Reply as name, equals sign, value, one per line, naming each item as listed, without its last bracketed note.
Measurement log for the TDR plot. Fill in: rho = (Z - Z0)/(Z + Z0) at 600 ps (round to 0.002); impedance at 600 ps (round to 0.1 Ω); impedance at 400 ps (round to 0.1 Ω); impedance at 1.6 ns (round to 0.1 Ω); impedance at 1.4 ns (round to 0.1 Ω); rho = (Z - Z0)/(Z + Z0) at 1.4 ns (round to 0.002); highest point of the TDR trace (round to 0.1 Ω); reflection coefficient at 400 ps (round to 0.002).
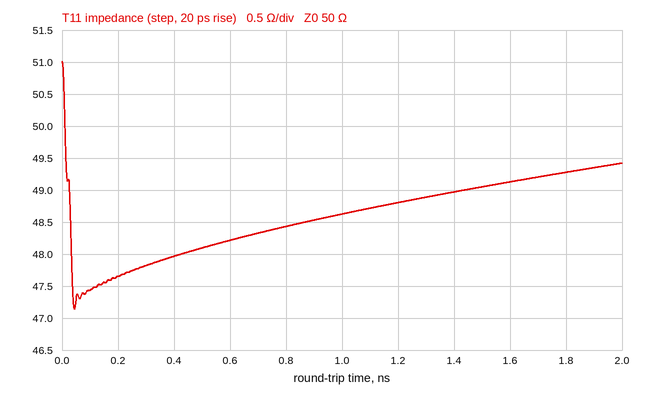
rho = (Z - Z0)/(Z + Z0) at 600 ps = -0.018
impedance at 600 ps = 48.2 Ω
impedance at 400 ps = 48.0 Ω
impedance at 1.6 ns = 49.1 Ω
impedance at 1.4 ns = 49.0 Ω
rho = (Z - Z0)/(Z + Z0) at 1.4 ns = -0.010
highest point of the TDR trace = 51.0 Ω
reflection coefficient at 400 ps = -0.020
